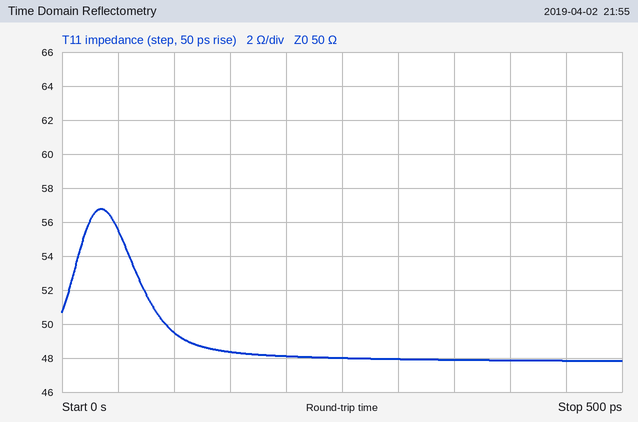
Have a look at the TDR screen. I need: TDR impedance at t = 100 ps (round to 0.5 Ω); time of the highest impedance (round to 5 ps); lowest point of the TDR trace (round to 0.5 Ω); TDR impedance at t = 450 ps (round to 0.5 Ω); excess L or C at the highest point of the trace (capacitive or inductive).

49.5 Ω
35 ps
48.0 Ω
48.0 Ω
inductive
